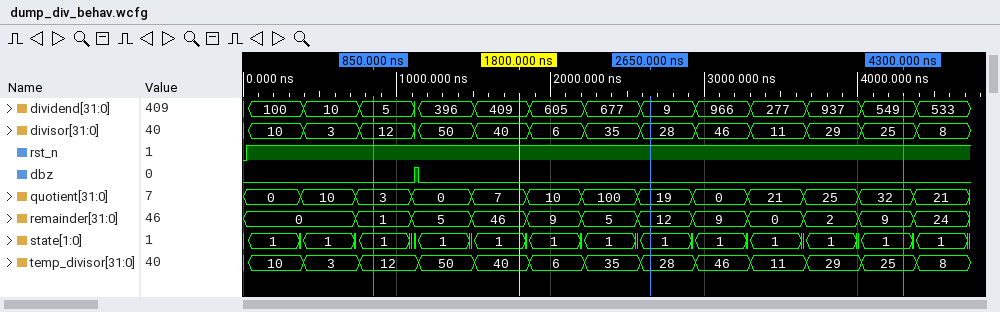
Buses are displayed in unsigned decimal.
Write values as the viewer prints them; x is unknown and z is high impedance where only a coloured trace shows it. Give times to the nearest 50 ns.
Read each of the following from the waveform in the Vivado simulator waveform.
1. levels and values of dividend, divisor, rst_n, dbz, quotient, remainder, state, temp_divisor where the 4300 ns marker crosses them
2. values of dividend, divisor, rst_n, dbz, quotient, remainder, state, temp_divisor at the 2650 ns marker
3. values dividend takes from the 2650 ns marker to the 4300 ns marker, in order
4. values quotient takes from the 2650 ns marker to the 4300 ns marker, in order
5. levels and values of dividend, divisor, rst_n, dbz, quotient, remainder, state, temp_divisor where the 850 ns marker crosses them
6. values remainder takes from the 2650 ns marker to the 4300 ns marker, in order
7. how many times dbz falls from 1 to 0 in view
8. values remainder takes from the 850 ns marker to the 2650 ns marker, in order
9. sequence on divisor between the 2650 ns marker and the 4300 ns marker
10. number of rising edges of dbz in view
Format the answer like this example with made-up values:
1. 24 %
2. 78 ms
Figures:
1. dividend=549, divisor=25, rst_n=1, dbz=0, quotient=32, remainder=9, state=1, temp_divisor=25
2. dividend=9, divisor=28, rst_n=1, dbz=0, quotient=19, remainder=12, state=1, temp_divisor=28
3. 9, 966, 277, 937, 549
4. 19, 0, 21, 25, 32
5. dividend=5, divisor=12, rst_n=1, dbz=0, quotient=3, remainder=1, state=1, temp_divisor=12
6. 12, 9, 0, 2, 9
7. 1
8. 1, 5, 46, 9, 5, 12
9. 28, 46, 11, 29, 25
10. 1
